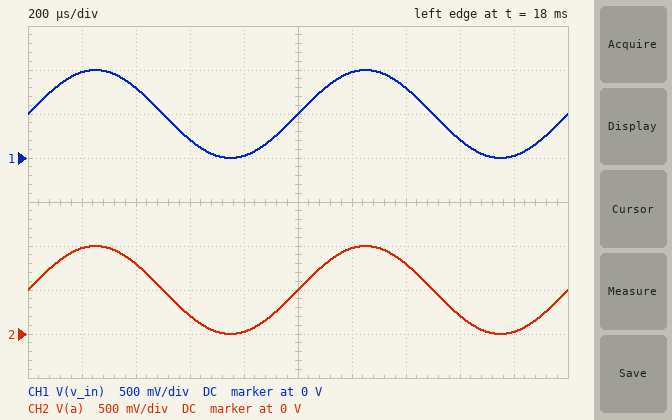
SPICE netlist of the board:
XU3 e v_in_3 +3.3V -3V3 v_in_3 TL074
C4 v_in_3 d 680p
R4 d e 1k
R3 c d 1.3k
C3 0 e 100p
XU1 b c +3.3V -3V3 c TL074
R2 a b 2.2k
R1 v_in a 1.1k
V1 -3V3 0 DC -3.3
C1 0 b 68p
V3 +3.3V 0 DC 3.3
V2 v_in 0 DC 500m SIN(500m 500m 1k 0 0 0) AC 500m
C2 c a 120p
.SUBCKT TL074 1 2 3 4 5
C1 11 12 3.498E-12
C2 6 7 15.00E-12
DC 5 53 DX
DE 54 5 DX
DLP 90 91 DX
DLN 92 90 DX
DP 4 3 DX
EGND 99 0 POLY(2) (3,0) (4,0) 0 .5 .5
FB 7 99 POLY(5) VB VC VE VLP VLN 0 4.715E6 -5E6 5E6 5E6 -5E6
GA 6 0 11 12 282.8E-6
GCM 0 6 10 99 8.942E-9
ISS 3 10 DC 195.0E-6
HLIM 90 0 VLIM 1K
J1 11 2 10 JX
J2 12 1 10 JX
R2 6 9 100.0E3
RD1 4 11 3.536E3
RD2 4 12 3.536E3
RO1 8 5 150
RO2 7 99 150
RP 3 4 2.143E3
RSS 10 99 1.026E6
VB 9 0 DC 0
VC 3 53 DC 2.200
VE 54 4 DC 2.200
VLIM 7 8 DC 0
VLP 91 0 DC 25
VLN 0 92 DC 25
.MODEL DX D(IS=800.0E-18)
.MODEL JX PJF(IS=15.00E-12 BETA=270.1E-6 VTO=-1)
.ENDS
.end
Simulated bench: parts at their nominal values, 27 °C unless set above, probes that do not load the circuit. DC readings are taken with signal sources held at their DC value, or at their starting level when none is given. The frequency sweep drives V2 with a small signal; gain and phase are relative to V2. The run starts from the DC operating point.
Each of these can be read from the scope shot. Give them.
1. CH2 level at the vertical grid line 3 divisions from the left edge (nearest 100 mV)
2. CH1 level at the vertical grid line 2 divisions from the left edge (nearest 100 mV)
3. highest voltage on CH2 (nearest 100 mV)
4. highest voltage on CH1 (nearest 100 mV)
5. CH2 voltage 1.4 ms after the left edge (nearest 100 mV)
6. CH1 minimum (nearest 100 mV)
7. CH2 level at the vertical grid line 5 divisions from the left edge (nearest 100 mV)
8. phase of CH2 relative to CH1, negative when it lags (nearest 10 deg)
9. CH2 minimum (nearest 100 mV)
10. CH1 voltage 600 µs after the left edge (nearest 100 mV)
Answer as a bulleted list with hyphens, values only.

- 200 mV
- 800 mV
- 1.0 V
- 1.0 V
- 800 mV
- 0 V
- 500 mV
- 0 deg
- 0 V
- 200 mV
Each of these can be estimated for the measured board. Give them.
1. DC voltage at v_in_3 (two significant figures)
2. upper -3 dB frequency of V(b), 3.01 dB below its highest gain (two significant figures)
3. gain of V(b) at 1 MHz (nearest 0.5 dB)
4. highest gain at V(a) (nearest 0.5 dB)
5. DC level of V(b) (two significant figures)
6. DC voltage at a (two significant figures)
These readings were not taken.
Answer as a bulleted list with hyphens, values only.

- 500 mV
- 970 kHz
- -3.5 dB
- 1.0 dB
- 500 mV
- 500 mV
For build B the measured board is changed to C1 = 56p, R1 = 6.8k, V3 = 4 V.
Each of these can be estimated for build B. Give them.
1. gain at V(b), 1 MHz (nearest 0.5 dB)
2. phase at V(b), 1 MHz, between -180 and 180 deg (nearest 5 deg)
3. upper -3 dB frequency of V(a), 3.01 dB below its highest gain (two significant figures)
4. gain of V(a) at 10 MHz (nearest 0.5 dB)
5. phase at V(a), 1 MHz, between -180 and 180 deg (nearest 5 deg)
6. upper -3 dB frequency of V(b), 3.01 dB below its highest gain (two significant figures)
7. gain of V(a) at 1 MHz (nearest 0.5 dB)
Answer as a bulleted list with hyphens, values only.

- -15.5 dB
- -145 deg
- 470 kHz
- -32.0 dB
- -105 deg
- 450 kHz
- -13.5 dB
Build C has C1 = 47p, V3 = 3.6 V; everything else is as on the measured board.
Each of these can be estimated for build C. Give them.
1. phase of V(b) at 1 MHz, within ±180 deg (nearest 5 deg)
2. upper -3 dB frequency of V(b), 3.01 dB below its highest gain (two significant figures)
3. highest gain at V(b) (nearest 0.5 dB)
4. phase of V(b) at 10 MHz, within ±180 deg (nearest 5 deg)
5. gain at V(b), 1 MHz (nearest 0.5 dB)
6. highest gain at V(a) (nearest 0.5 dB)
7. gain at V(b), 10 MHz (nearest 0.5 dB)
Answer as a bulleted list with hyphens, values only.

- -80 deg
- 1.2 MHz
- 1.0 dB
- -110 deg
- -0.5 dB
- 1.5 dB
- -33.5 dB
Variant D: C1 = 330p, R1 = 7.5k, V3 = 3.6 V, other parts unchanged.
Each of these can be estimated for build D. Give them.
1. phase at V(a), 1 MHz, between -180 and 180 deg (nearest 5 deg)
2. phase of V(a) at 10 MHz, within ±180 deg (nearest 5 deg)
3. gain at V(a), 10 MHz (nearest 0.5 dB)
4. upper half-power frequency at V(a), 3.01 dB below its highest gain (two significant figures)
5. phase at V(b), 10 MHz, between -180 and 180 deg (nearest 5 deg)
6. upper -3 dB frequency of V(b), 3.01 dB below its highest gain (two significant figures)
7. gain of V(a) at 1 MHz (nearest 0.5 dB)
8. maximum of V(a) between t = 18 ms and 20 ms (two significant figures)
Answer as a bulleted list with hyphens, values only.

- -65 deg
- -35 deg
- -32.5 dB
- 57 kHz
- -120 deg
- 53 kHz
- -17.5 dB
- 1.0 V
